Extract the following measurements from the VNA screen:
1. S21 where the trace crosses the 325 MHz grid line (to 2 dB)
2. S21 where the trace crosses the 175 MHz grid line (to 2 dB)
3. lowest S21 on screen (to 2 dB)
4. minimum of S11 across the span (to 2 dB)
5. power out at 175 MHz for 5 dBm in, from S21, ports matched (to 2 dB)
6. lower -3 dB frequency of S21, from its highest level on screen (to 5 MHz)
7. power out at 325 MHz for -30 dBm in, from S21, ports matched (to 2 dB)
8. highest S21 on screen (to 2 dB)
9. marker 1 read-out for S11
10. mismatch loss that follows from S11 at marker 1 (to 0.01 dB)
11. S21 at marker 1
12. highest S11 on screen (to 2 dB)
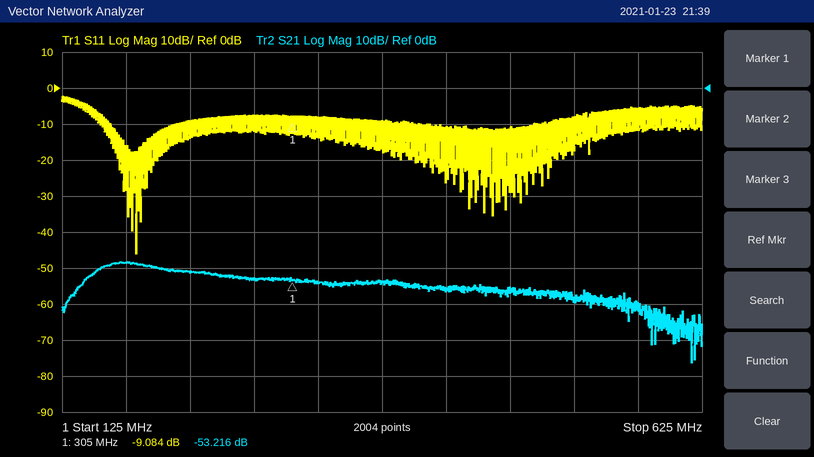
-54 dB
-48 dB
-76 dB
-46 dB
-44 dBm
150 MHz
-84 dBm
-48 dB
-9.084 dB
0.57 dB
-53.216 dB
-2 dB
